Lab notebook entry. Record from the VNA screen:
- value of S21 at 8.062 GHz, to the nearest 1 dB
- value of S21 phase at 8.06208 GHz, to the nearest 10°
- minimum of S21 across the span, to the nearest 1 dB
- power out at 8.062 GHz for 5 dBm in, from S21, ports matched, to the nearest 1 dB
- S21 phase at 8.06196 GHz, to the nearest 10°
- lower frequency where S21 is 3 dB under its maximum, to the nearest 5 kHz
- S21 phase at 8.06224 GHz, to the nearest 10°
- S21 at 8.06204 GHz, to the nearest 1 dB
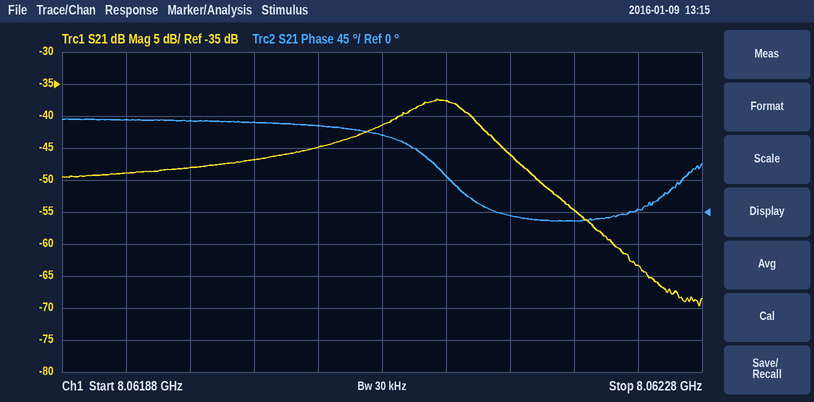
-47 dB
110°
-70 dB
-42 dBm
130°
8.062090 GHz
0°
-45 dB
